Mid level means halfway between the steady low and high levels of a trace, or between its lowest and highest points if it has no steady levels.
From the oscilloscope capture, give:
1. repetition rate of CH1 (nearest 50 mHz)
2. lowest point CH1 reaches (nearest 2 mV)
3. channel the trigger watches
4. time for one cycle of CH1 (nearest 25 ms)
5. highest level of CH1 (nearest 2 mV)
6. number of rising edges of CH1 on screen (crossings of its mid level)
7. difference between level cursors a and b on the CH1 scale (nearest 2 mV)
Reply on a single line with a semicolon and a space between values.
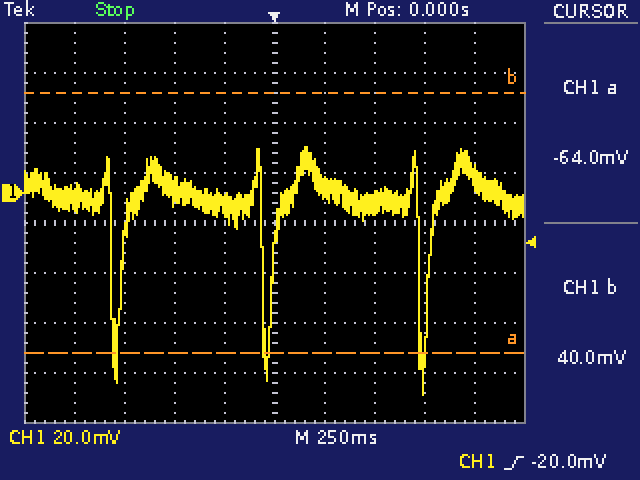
1.30 Hz; -80 mV; CH1; 775 ms; 18 mV; 3; 104 mV
